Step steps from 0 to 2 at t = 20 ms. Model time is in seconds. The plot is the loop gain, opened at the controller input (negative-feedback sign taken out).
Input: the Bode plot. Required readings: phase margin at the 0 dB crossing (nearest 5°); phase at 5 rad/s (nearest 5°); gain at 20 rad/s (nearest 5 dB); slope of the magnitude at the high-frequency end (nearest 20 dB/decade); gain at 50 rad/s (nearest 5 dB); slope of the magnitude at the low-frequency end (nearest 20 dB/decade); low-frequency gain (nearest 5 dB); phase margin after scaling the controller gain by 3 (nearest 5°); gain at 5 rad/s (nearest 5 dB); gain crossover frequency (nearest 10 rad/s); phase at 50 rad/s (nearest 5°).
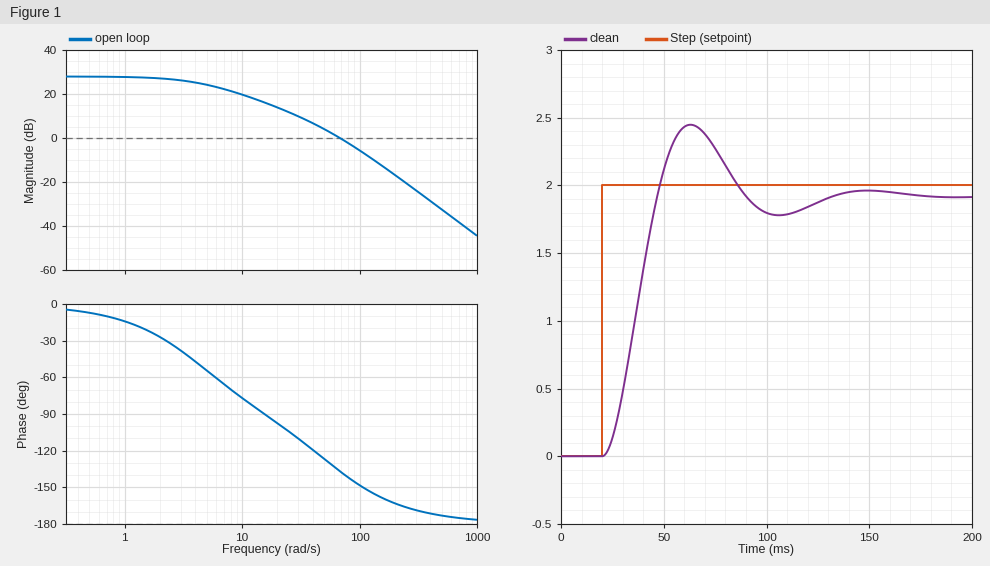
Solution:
45°
-55°
15 dB
-40 dB/decade
5 dB
0 dB/decade
30 dB
25°
25 dB
70 rad/s
-125°
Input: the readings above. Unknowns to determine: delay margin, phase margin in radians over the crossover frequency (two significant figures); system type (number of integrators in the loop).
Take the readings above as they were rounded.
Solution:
0.011 s
0
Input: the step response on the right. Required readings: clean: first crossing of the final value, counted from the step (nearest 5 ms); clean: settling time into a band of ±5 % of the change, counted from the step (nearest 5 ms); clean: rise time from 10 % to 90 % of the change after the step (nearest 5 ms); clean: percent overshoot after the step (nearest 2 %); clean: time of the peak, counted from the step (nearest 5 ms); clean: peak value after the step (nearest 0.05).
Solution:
25 ms
100 ms
20 ms
28 %
45 ms
2.45
